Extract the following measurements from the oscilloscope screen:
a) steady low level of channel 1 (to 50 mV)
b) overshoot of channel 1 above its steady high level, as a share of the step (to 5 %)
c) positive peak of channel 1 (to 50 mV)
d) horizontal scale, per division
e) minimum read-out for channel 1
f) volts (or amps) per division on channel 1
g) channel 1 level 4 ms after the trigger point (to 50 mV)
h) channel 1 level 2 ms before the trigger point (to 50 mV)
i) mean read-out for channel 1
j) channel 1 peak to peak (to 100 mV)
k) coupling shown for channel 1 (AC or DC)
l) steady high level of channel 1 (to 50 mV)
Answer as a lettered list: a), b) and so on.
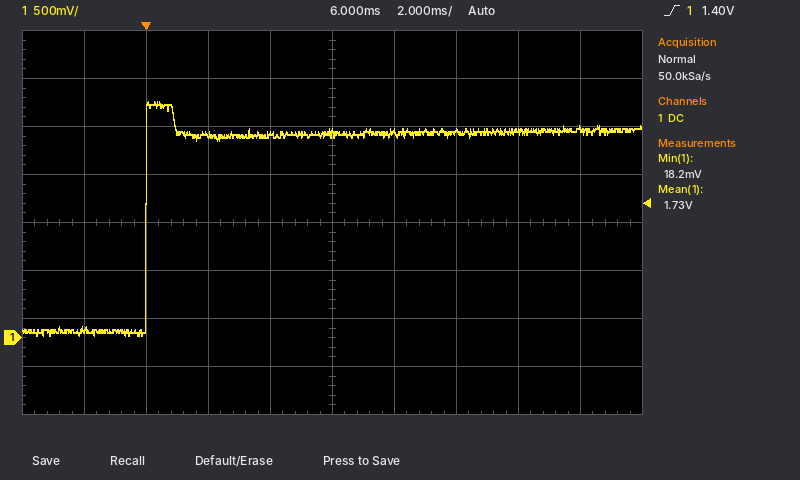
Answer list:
a) 50 mV
b) 15 %
c) 2.45 V
d) 2 ms
e) 18.2 mV
f) 500 mV
g) 2.10 V
h) 100 mV
i) 1.73 V
j) 2.40 V
k) DC
l) 2.15 V
